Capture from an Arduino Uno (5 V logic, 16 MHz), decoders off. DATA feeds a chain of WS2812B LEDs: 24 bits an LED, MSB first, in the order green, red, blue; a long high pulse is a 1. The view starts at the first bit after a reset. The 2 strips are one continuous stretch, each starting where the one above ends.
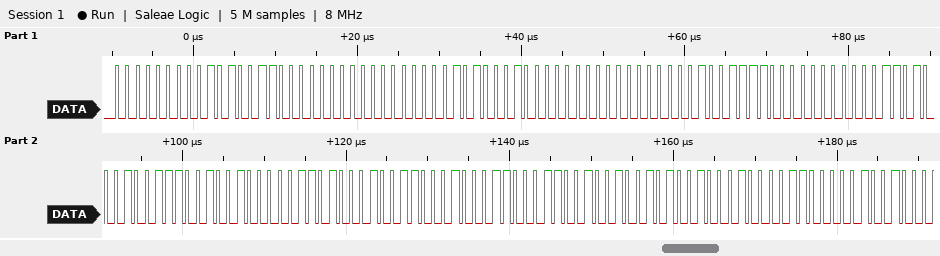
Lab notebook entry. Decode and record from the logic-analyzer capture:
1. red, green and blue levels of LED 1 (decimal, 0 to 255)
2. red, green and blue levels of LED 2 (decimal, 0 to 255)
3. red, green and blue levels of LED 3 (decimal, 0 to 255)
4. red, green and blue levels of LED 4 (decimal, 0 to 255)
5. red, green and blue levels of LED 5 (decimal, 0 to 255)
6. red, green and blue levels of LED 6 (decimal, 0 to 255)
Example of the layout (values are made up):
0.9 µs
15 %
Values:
83, 0, 0
81, 0, 0
79, 0, 0
39, 26, 36
38, 26, 35
37, 25, 34
